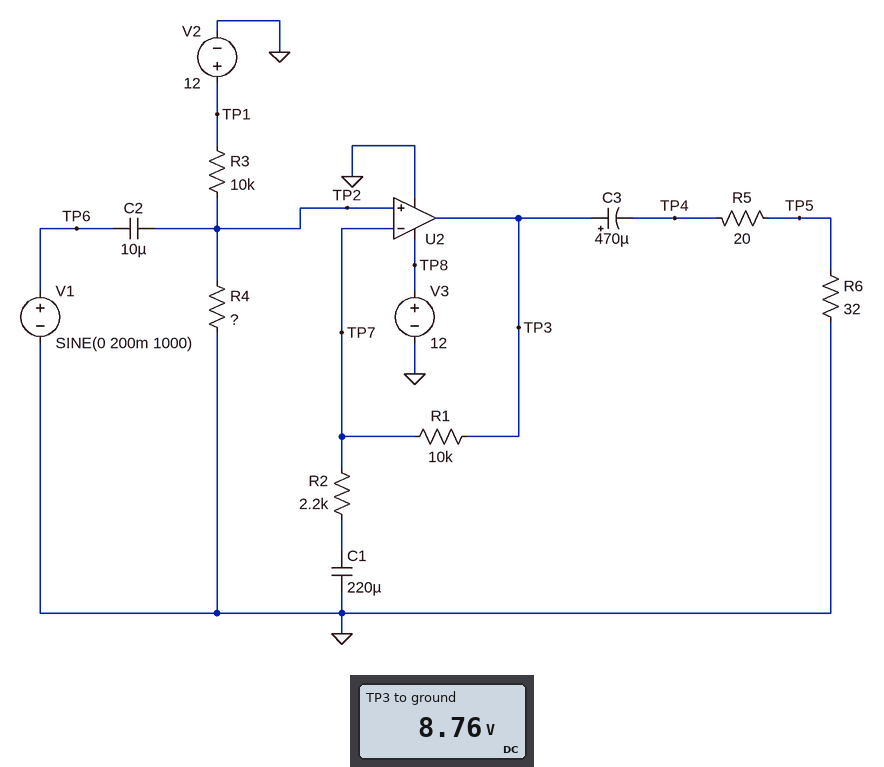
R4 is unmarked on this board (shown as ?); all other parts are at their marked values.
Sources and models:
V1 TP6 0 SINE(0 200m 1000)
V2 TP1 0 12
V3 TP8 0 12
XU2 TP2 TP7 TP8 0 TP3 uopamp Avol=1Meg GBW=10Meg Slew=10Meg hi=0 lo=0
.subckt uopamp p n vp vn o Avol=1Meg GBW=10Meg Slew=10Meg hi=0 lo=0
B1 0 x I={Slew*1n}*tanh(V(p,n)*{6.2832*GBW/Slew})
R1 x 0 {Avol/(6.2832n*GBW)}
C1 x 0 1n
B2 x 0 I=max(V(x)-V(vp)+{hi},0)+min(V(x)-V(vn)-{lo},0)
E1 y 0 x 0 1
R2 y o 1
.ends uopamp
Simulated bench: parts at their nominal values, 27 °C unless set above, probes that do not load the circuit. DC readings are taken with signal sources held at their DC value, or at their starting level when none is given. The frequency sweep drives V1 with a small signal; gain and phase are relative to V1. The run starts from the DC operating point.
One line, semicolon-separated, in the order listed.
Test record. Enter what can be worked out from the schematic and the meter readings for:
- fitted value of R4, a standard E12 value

27 kΩ
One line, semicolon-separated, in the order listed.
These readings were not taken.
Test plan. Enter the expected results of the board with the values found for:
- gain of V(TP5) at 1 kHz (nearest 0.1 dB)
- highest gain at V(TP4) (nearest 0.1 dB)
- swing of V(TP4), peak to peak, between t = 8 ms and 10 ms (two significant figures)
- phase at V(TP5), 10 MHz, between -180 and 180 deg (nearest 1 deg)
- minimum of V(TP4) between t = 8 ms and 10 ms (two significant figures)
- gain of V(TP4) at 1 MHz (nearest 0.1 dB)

10.7 dB; 14.9 dB; 2.2 V; -80 deg; -1.1 V; 13.7 dB
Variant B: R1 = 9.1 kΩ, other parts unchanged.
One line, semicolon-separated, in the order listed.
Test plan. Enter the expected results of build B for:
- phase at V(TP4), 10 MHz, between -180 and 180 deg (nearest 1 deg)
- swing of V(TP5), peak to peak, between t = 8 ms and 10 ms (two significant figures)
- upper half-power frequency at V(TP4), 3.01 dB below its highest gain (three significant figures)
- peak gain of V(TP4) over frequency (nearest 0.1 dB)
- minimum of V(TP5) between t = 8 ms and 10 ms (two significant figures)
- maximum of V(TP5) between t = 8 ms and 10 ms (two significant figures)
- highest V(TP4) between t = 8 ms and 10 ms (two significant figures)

-79 deg; 1.3 V; 1.91 MHz; 14.2 dB; -640 mV; 630 mV; 1.0 V
